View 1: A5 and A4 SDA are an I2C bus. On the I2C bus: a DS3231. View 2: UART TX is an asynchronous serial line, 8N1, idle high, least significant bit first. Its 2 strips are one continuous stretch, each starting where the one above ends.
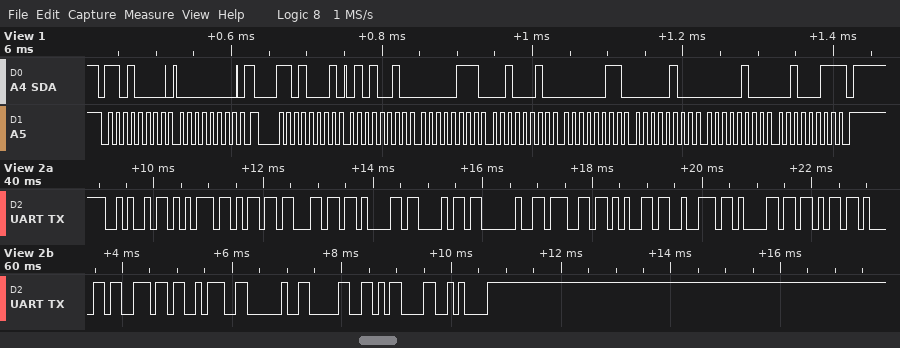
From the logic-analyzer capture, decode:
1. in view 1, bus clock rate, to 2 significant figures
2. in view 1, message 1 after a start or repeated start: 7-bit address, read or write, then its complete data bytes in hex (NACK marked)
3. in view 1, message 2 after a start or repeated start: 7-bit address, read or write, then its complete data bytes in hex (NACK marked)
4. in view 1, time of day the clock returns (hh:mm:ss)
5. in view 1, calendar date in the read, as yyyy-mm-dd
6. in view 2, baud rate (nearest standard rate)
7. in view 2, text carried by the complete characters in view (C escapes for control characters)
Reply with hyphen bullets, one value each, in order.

- 100 kHz
- 0x68 write: 00
- 0x68 read: 52 07 22 03 04 04 23 NACK
- 22:07:52
- 2023-04-04
- 9600 baud
- "Jumlah gerakan: 0\r\n"
